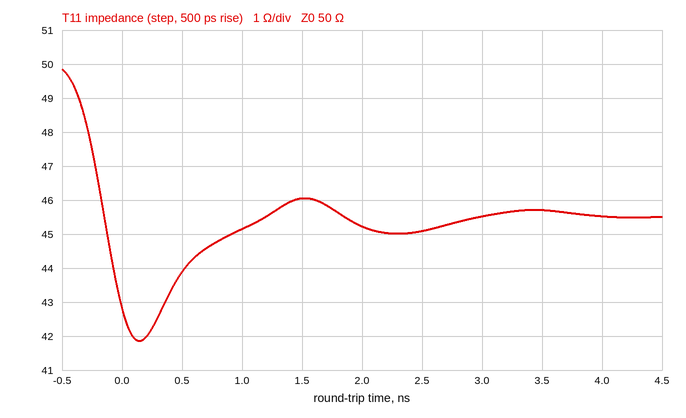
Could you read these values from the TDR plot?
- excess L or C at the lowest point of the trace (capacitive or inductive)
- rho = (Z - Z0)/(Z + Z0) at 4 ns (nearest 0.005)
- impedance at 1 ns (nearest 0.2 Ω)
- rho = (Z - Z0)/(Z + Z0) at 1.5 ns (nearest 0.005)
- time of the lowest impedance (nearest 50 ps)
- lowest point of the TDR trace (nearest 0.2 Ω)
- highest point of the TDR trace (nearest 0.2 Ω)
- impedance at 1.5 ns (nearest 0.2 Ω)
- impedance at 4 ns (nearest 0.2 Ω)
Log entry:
capacitive
-0.045
45.2 Ω
-0.040
150 ps
41.8 Ω
49.8 Ω
46.0 Ω
45.6 Ω
